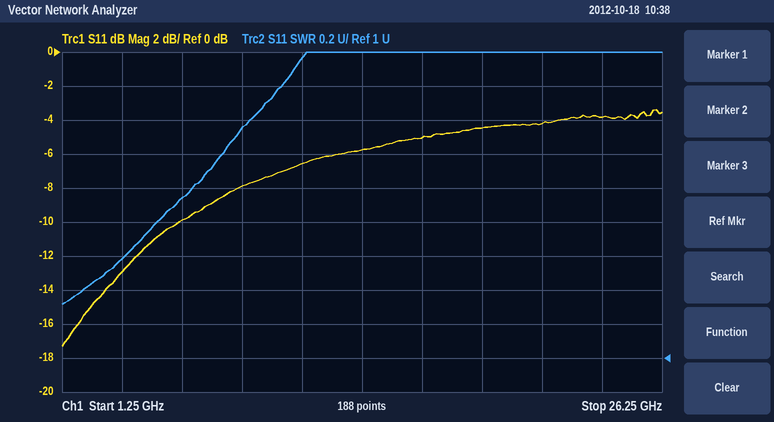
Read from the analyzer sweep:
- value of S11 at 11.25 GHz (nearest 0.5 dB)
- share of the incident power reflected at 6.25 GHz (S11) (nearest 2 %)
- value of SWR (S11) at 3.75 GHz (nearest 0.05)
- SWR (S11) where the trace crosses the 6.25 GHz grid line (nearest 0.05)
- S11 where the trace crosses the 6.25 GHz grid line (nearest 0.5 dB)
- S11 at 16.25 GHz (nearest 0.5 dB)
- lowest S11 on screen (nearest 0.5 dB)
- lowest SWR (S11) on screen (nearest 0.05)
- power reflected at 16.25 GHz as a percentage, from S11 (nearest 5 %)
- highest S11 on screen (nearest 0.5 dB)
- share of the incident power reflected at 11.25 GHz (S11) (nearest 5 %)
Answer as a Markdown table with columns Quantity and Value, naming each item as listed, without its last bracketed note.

| Quantity | Value |
|---|---|
| value of S11 at 11.25 GHz | -6.5 dB |
| share of the incident power reflected at 6.25 GHz (S11) | 10 % |
| value of SWR (S11) at 3.75 GHz | 1.60 |
| SWR (S11) where the trace crosses the 6.25 GHz grid line | 1.95 |
| S11 where the trace crosses the 6.25 GHz grid line | -10.0 dB |
| S11 at 16.25 GHz | -5.0 dB |
| lowest S11 on screen | -17.5 dB |
| lowest SWR (S11) on screen | 1.30 |
| power reflected at 16.25 GHz as a percentage, from S11 | 30 % |
| highest S11 on screen | -3.5 dB |
| share of the incident power reflected at 11.25 GHz (S11) | 20 % |
